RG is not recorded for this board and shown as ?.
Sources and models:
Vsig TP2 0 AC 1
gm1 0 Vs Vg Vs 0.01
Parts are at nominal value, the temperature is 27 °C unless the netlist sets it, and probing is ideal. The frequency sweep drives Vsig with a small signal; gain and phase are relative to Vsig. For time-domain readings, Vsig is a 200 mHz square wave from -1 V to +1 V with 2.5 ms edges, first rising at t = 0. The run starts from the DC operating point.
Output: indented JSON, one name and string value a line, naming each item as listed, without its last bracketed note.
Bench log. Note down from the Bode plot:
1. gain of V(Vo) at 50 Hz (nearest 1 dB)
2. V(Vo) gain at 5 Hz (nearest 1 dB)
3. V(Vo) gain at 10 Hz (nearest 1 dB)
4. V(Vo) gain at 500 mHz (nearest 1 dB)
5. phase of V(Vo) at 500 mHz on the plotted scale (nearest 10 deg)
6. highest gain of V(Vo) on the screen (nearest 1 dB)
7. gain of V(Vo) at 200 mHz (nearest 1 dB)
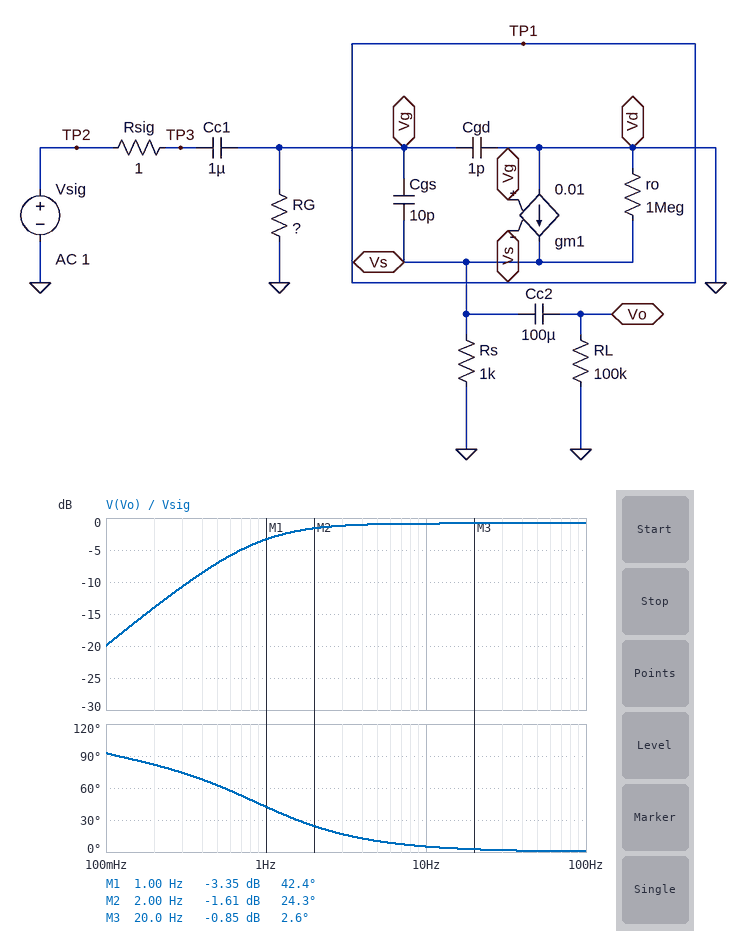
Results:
{
  "gain of V(Vo) at 50 Hz": "-1 dB",
  "V(Vo) gain at 5 Hz": "-1 dB",
  "V(Vo) gain at 10 Hz": "-1 dB",
  "V(Vo) gain at 500 mHz": "-7 dB",
  "phase of V(Vo) at 500 mHz on the plotted scale": "60 deg",
  "highest gain of V(Vo) on the screen": "-1 dB",
  "gain of V(Vo) at 200 mHz": "-14 dB"
}
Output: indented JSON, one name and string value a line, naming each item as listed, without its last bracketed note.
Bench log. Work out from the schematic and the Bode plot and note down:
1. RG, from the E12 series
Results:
{
  "RG, from the E12 series": "180 kΩ"
}
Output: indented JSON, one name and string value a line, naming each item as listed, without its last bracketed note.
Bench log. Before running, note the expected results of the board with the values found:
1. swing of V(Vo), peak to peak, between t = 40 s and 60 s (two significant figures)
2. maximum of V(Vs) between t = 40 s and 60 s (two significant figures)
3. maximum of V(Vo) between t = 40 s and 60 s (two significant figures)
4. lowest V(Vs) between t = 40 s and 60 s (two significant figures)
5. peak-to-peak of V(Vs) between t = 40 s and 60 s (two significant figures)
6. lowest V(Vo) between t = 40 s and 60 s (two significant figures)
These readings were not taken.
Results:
{
  "swing of V(Vo), peak to peak, between t = 40 s and 60 s": "3.6 V",
  "maximum of V(Vs) between t = 40 s and 60 s": "1.8 V",
  "maximum of V(Vo) between t = 40 s and 60 s": "1.8 V",
  "lowest V(Vs) between t = 40 s and 60 s": "-1.8 V",
  "peak-to-peak of V(Vs) between t = 40 s and 60 s": "3.6 V",
  "lowest V(Vo) between t = 40 s and 60 s": "-1.8 V"
}
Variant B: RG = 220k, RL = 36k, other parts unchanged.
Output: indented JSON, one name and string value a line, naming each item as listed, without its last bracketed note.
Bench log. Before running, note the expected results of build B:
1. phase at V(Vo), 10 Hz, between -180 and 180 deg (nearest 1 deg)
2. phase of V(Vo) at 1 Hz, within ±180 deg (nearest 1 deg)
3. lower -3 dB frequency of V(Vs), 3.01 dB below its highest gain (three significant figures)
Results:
{
  "phase at V(Vo), 10 Hz, between -180 and 180 deg": "4 deg",
  "phase of V(Vo) at 1 Hz, within ±180 deg": "38 deg",
  "lower -3 dB frequency of V(Vs), 3.01 dB below its highest gain": "723 mHz"
}
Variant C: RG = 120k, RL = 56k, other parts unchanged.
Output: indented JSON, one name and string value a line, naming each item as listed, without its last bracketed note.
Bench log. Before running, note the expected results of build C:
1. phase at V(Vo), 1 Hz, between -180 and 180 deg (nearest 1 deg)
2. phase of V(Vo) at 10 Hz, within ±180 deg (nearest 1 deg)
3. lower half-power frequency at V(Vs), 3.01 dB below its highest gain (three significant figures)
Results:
{
  "phase at V(Vo), 1 Hz, between -180 and 180 deg": "55 deg",
  "phase of V(Vo) at 10 Hz, within ±180 deg": "8 deg",
  "lower half-power frequency at V(Vs), 3.01 dB below its highest gain": "1.33 Hz"
}
